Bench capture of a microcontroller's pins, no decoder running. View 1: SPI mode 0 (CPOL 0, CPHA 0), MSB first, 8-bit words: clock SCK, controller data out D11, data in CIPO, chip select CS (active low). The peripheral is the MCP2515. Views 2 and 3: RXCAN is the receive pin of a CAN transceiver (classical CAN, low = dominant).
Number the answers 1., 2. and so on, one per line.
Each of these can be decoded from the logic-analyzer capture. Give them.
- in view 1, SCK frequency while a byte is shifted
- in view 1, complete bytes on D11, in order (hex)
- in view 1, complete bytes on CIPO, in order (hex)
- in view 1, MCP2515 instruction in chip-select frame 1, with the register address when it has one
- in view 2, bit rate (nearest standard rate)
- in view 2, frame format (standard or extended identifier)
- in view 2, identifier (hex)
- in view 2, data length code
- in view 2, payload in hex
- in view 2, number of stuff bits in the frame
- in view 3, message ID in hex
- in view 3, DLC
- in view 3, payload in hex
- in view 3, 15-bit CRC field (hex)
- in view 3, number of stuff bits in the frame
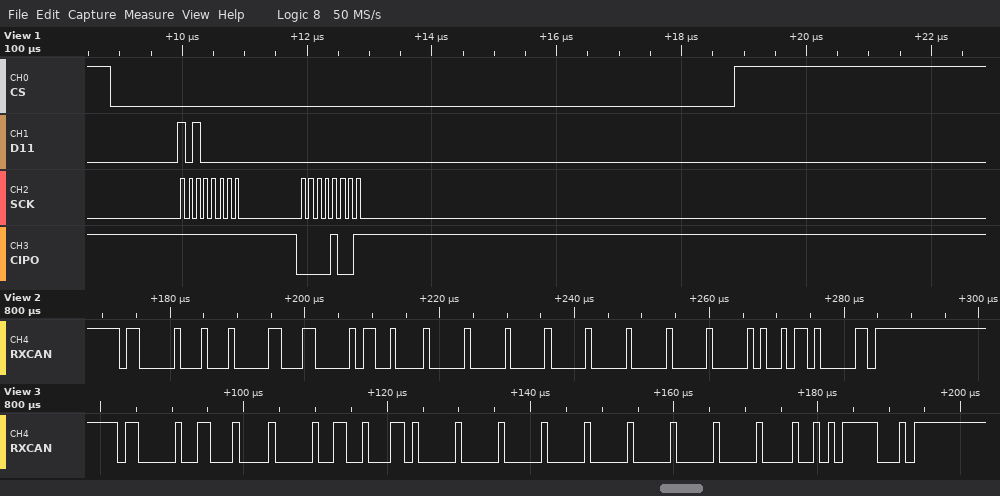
1. 8 MHz
2. A0 00
3. FF 09
4. READ STATUS
5. 1000 kbit/s
6. standard
7. 0x601
8. 8
9. 23 03 21 00 00 00 00 00
10. 12
11. 0x603
12. 8
13. 40 64 68 00 00 00 00 00
14. 0x257C
15. 11
